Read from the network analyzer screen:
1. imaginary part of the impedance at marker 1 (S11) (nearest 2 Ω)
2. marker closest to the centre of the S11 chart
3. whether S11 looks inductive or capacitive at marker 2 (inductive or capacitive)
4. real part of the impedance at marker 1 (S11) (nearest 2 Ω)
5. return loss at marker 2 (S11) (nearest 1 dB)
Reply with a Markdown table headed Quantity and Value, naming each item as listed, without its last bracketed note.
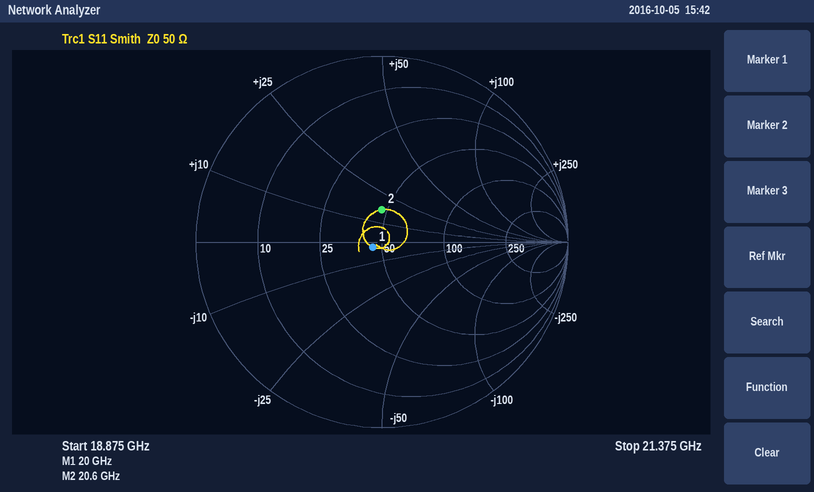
| Quantity | Value |
|---|---|
| imaginary part of the impedance at marker 1 (S11) | -2 Ω |
| marker closest to the centre of the S11 chart | marker 1 |
| whether S11 looks inductive or capacitive at marker 2 | inductive |
| real part of the impedance at marker 1 (S11) | 46 Ω |
| return loss at marker 2 (S11) | 15 dB |
